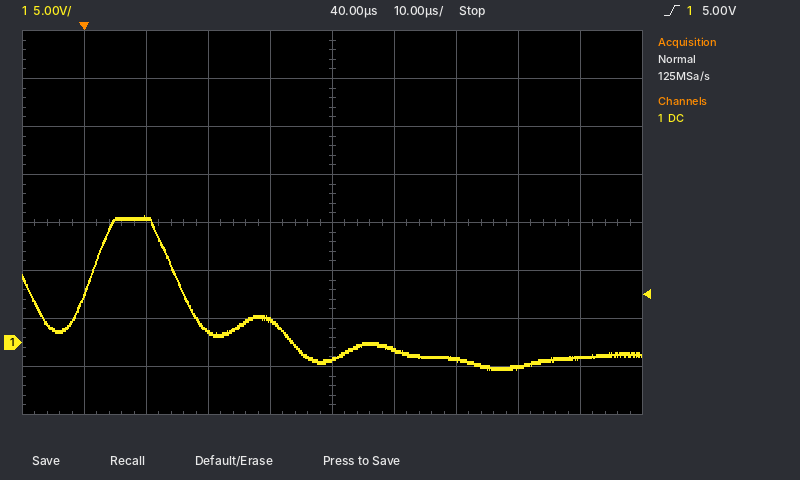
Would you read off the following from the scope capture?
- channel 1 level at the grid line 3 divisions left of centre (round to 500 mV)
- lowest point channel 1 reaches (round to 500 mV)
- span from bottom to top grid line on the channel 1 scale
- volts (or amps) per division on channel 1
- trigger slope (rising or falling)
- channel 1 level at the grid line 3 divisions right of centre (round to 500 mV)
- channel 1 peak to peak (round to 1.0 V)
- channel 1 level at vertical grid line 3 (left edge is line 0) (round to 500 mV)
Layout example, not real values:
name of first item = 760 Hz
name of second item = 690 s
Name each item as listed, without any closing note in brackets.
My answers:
channel 1 level at the grid line 3 divisions left of centre = 13.0 V
lowest point channel 1 reaches = -3.0 V
span from bottom to top grid line on the channel 1 scale = 40 V
volts (or amps) per division on channel 1 = 5 V
trigger slope = rising
channel 1 level at the grid line 3 divisions right of centre = -2.5 V
channel 1 peak to peak = 16.0 V
channel 1 level at vertical grid line 3 (left edge is line 0) = 1.0 V
